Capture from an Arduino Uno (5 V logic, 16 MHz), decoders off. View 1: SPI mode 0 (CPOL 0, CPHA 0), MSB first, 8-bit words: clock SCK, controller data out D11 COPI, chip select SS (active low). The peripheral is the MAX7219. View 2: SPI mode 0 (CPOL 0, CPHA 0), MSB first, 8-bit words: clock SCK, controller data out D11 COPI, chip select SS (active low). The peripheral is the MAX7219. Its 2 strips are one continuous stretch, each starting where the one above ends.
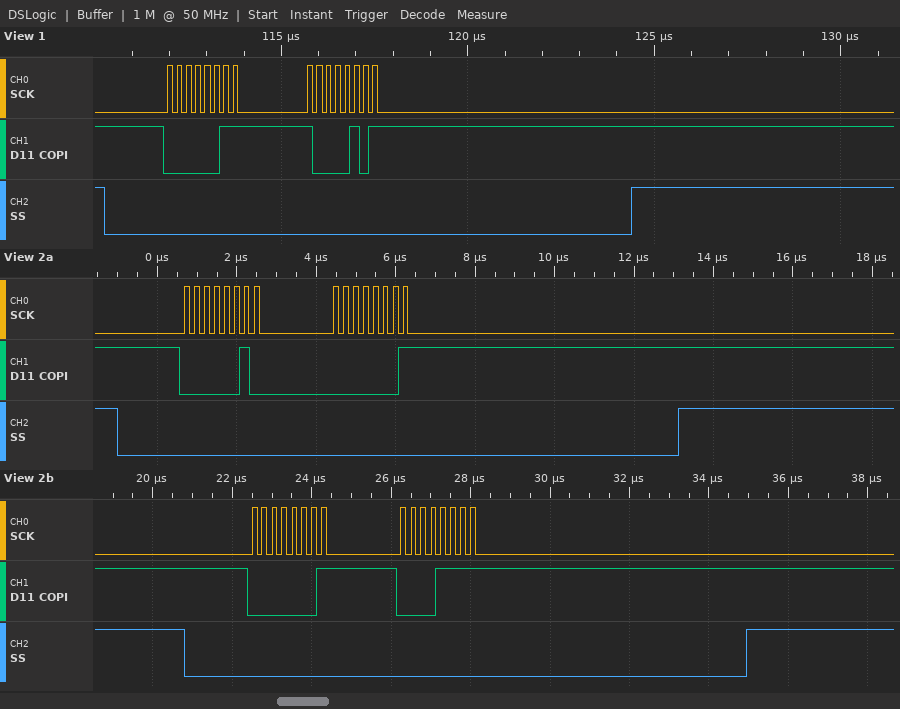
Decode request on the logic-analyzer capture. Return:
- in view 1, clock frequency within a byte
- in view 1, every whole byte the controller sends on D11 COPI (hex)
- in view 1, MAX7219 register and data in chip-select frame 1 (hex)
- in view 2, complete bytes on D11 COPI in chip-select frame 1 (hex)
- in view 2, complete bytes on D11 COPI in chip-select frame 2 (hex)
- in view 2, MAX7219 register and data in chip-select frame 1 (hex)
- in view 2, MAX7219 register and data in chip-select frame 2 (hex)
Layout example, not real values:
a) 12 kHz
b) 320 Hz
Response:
a) 4 MHz
b) 03 85
c) register 0x3, data 0x85
d) 02 01
e) 01 0F
f) register 0x2, data 0x01
g) register 0x1, data 0x0F
